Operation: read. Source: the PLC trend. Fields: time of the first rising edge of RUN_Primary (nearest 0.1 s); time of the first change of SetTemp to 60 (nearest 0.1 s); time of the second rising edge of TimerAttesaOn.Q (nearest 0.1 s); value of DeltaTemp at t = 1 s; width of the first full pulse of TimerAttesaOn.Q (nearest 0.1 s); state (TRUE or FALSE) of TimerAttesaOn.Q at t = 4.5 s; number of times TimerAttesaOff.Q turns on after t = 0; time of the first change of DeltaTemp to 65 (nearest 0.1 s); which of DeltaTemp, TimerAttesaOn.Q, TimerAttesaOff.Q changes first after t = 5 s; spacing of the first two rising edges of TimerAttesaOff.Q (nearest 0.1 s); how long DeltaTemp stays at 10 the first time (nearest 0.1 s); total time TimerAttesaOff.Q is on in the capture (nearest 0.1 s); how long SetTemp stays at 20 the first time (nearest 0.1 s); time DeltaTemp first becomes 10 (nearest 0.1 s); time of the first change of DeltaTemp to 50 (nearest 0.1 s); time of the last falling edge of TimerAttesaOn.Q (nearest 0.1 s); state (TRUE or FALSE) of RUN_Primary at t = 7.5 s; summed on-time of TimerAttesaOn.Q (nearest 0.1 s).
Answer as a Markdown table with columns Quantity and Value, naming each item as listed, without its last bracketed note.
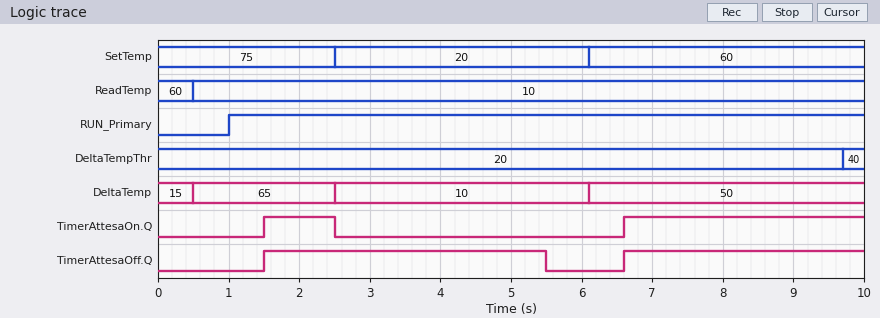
| Quantity | Value |
|---|---|
| time of the first rising edge of RUN_Primary | 1.0 s |
| time of the first change of SetTemp to 60 | 6.1 s |
| time of the second rising edge of TimerAttesaOn.Q | 6.6 s |
| value of DeltaTemp at t = 1 s | 65 |
| width of the first full pulse of TimerAttesaOn.Q | 1.0 s |
| state (TRUE or FALSE) of TimerAttesaOn.Q at t = 4.5 s | FALSE |
| number of times TimerAttesaOff.Q turns on after t = 0 | 2 |
| time of the first change of DeltaTemp to 65 | 0.5 s |
| which of DeltaTemp, TimerAttesaOn.Q, TimerAttesaOff.Q changes first after t = 5 s | TimerAttesaOff.Q |
| spacing of the first two rising edges of TimerAttesaOff.Q | 5.1 s |
| how long DeltaTemp stays at 10 the first time | 3.6 s |
| total time TimerAttesaOff.Q is on in the capture | 7.4 s |
| how long SetTemp stays at 20 the first time | 3.6 s |
| time DeltaTemp first becomes 10 | 2.5 s |
| time of the first change of DeltaTemp to 50 | 6.1 s |
| time of the last falling edge of TimerAttesaOn.Q | 2.5 s |
| state (TRUE or FALSE) of RUN_Primary at t = 7.5 s | TRUE |
| summed on-time of TimerAttesaOn.Q | 4.4 s |
